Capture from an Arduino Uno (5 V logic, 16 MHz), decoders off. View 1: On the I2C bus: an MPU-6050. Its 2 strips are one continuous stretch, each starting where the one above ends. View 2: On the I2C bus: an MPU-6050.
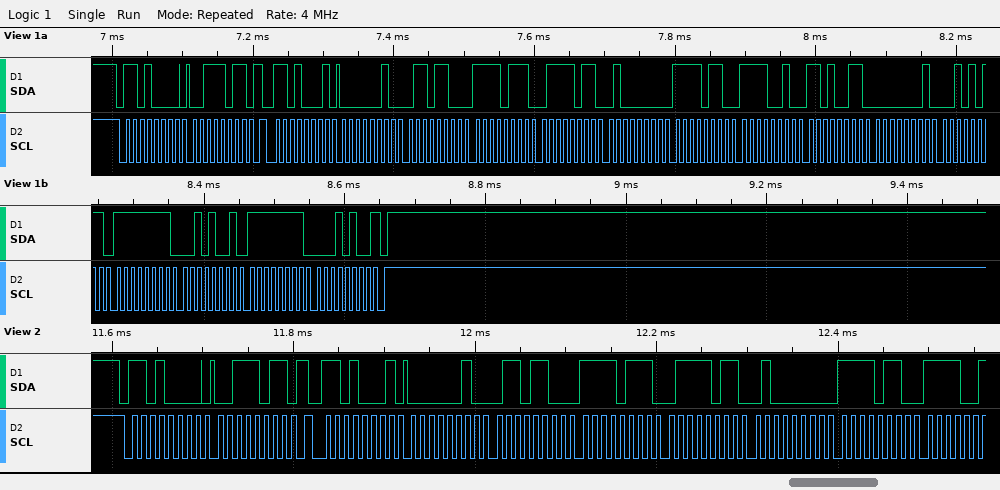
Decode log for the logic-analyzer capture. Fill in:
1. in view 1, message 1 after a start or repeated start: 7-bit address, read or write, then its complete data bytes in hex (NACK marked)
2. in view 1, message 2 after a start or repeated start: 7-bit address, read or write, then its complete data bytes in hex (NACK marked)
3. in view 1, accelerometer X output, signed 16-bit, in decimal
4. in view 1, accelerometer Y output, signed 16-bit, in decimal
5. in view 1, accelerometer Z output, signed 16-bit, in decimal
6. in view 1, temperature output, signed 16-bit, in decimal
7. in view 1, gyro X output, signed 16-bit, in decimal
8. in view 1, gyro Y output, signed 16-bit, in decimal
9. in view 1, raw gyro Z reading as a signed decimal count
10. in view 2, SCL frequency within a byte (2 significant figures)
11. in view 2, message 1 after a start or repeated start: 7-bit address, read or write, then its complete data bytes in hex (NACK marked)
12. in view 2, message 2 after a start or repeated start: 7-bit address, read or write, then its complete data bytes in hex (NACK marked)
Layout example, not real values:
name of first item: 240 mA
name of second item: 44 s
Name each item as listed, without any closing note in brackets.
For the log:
in view 1, message 1 after a start or repeated start: 7-bit address, read or write, then its complete data bytes in hex: 0x68 write: 3B
in view 1, message 2 after a start or repeated start: 7-bit address, read or write, then its complete data bytes in hex: 0x68 read: 02 6C F7 7B 40 F6 F2 D3 01 2B FF 29 FF 14 NACK
in view 1, accelerometer X output, signed 16-bit, in decimal: 620
in view 1, accelerometer Y output, signed 16-bit, in decimal: -2181
in view 1, accelerometer Z output, signed 16-bit, in decimal: 16630
in view 1, temperature output, signed 16-bit, in decimal: -3373
in view 1, gyro X output, signed 16-bit, in decimal: 299
in view 1, gyro Y output, signed 16-bit, in decimal: -215
in view 1, raw gyro Z reading as a signed decimal count: -236
in view 2, SCL frequency within a byte: 100 kHz
in view 2, message 1 after a start or repeated start: 7-bit address, read or write, then its complete data bytes in hex: 0x68 write: 3B
in view 2, message 2 after a start or repeated start: 7-bit address, read or write, then its complete data bytes in hex: 0x68 read: 02 6C F7 7B 40 F6
